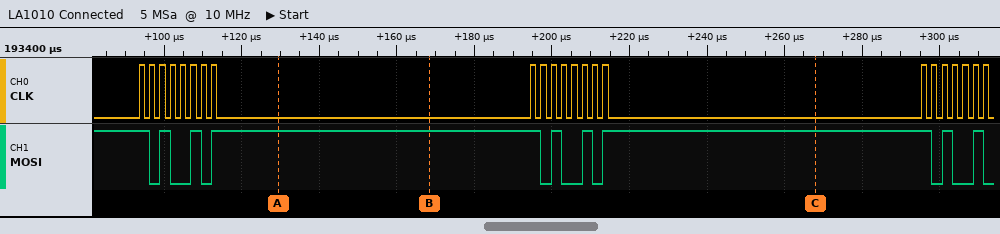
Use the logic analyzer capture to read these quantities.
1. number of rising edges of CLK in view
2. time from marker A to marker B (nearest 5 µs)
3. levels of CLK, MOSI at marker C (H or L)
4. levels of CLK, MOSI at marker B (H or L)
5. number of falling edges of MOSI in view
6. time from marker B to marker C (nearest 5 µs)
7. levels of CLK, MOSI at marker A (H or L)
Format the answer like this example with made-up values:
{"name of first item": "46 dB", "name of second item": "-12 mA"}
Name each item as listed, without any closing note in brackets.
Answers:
{"number of rising edges of CLK in view": "23", "time from marker A to marker B": "40 µs", "levels of CLK, MOSI at marker C": "CLK=L, MOSI=H", "levels of CLK, MOSI at marker B": "CLK=L, MOSI=H", "number of falling edges of MOSI in view": "9", "time from marker B to marker C": "100 µs", "levels of CLK, MOSI at marker A": "CLK=L, MOSI=H"}
